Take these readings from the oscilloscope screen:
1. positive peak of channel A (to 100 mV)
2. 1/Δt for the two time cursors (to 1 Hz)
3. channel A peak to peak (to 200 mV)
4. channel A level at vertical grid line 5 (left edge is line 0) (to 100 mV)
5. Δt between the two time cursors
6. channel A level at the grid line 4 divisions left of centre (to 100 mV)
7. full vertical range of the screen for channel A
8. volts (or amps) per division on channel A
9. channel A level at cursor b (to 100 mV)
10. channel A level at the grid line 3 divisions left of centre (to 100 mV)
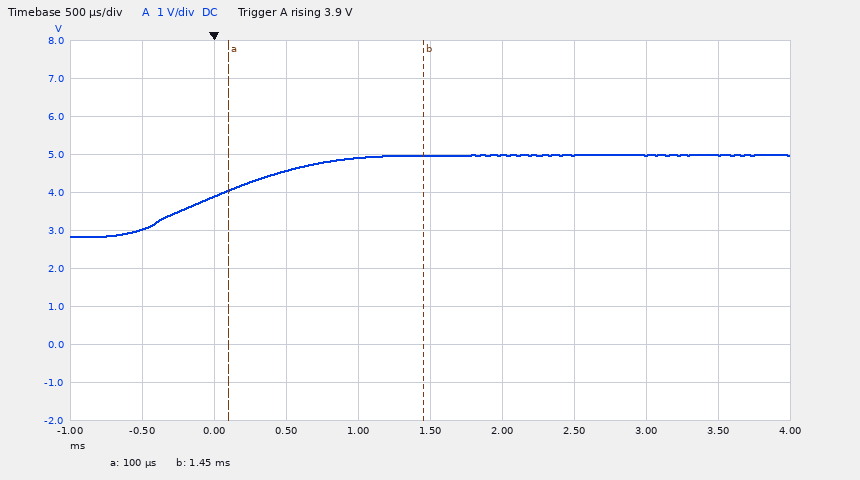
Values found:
5.0 V
741 Hz
2.2 V
5.0 V
1.35 ms
3.0 V
10 V
1 V
5.0 V
3.9 V
